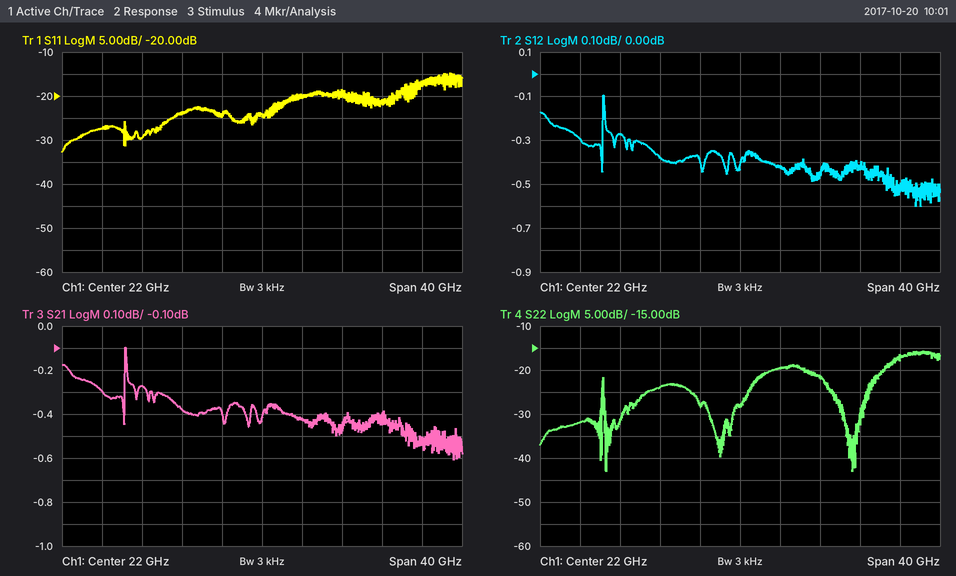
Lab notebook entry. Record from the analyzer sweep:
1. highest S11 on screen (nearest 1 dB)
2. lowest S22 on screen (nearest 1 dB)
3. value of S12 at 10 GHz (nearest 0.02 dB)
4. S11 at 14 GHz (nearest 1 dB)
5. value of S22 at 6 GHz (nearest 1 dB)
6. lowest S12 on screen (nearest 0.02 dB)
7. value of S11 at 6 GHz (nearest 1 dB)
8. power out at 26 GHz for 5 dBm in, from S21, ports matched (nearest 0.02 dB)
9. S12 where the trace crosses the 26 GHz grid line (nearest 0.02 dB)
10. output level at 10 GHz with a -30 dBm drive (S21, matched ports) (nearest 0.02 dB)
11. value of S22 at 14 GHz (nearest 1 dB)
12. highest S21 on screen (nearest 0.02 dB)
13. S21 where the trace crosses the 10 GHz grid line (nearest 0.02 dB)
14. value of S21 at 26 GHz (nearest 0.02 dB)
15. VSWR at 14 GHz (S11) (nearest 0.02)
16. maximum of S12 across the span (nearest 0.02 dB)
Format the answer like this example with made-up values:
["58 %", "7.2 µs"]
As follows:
["-15 dB", "-43 dB", "-0.28 dB", "-24 dB", "-32 dB", "-0.60 dB", "-27 dB", "4.58 dBm", "-0.42 dB", "-30.28 dBm", "-24 dB", "-0.10 dB", "-0.28 dB", "-0.42 dB", "1.14", "-0.10 dB"]
